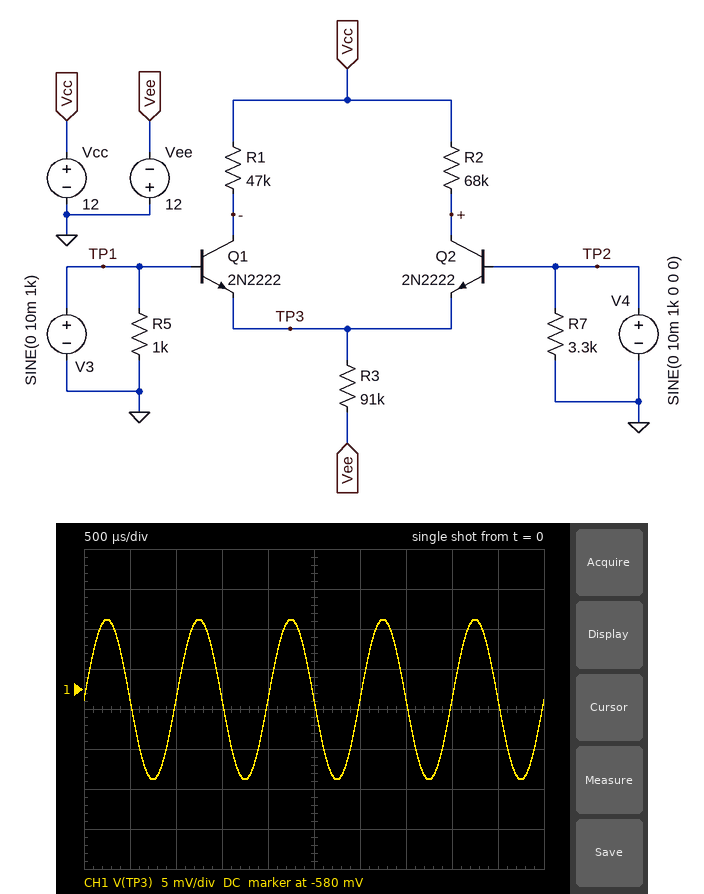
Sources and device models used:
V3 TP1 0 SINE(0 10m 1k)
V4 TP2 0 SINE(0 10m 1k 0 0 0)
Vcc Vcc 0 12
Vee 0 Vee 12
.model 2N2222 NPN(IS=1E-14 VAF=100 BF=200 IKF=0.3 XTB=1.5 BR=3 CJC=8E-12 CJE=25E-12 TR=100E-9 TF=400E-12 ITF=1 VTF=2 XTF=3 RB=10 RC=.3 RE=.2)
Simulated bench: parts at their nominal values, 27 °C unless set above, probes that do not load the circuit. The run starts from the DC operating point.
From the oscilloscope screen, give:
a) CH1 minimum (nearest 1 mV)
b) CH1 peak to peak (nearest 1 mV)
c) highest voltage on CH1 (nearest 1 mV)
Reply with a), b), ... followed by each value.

a) -591 mV
b) 20 mV
c) -571 mV
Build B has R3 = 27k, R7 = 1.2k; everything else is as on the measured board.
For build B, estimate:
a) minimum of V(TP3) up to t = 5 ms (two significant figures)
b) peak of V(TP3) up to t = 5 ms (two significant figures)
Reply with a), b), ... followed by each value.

a) -630 mV
b) -610 mV
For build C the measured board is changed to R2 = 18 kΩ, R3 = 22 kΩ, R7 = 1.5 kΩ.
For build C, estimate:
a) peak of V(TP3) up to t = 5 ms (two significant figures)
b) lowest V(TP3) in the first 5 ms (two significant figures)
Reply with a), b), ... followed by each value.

a) -610 mV
b) -630 mV
